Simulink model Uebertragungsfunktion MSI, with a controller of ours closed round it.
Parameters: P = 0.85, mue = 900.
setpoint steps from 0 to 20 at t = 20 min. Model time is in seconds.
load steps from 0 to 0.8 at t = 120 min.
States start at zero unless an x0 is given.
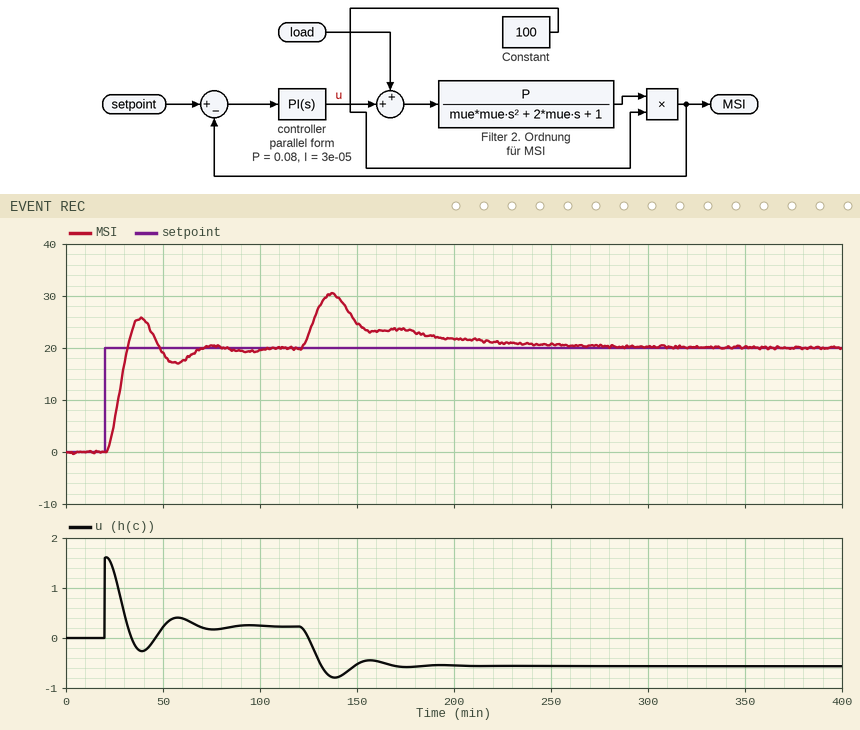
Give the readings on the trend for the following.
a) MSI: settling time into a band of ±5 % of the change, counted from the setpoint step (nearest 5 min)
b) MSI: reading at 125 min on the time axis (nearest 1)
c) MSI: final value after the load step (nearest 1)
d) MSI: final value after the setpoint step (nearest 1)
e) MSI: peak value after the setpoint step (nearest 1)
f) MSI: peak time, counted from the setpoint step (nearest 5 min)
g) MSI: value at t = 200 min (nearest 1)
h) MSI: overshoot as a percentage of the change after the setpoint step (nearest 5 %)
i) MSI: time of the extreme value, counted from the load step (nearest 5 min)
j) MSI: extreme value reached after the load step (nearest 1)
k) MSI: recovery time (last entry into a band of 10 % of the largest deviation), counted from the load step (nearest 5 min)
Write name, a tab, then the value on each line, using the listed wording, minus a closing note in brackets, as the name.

MSI: settling time into a band of ±5 % of the change, counted from the setpoint step	45 min
MSI: reading at 125 min on the time axis	23
MSI: final value after the load step	20
MSI: final value after the setpoint step	20
MSI: peak value after the setpoint step	26
MSI: peak time, counted from the setpoint step	20 min
MSI: value at t = 200 min	22
MSI: overshoot as a percentage of the change after the setpoint step	30 %
MSI: time of the extreme value, counted from the load step	15 min
MSI: extreme value reached after the load step	30
MSI: recovery time (last entry into a band of 10 % of the largest deviation), counted from the load step	105 min
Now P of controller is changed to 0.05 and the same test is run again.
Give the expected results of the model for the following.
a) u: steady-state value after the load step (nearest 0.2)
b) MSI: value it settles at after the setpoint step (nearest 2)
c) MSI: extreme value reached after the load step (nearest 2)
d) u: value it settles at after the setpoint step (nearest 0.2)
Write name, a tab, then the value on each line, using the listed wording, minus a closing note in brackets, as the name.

u: steady-state value after the load step	-0.6
MSI: value it settles at after the setpoint step	20
MSI: extreme value reached after the load step	34
u: value it settles at after the setpoint step	0.2
